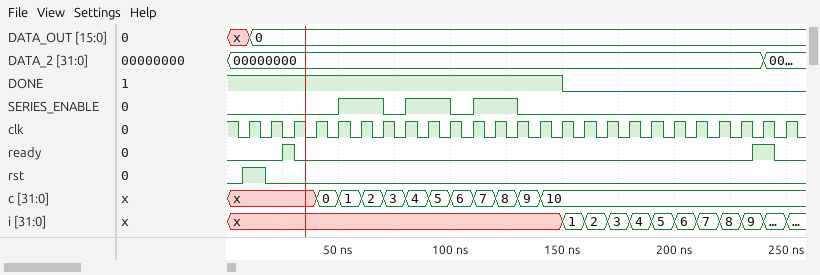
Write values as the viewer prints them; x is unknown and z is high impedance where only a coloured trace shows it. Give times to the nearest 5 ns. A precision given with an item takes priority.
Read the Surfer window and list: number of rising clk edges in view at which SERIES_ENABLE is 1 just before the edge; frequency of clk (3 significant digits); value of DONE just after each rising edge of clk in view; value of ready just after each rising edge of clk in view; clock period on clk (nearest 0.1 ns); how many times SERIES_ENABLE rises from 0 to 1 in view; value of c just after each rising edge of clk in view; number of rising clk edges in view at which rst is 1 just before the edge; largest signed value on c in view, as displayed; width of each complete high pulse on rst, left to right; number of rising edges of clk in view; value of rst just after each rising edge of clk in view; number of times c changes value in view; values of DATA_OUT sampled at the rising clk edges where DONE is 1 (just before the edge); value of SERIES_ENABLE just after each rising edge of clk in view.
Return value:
6
100 MHz
1 1 1 1 1 1 1 1 1 1 1 1 1 1 0 0 0 0 0 0 0 0 0 0 0
0 0 0 0 0 0 0 0 0 0 0 0 0 0 0 0 0 0 0 0 0 0 0 1 0
10 ns
3
x, x, x, 0, 1, 2, 3, 4, 5, 6, 7, 8, 9, 10, 10, 10, 10, 10, 10, 10, 10, 10, 10, 10, 10
1
10
10 ns
25
1 0 0 0 0 0 0 0 0 0 0 0 0 0 0 0 0 0 0 0 0 0 0 0 0
11
x, 0, 0, 0, 0, 0, 0, 0, 0, 0, 0, 0, 0, 0, 0
0 0 0 0 1 1 0 1 1 0 1 1 0 0 0 0 0 0 0 0 0 0 0 0 0
